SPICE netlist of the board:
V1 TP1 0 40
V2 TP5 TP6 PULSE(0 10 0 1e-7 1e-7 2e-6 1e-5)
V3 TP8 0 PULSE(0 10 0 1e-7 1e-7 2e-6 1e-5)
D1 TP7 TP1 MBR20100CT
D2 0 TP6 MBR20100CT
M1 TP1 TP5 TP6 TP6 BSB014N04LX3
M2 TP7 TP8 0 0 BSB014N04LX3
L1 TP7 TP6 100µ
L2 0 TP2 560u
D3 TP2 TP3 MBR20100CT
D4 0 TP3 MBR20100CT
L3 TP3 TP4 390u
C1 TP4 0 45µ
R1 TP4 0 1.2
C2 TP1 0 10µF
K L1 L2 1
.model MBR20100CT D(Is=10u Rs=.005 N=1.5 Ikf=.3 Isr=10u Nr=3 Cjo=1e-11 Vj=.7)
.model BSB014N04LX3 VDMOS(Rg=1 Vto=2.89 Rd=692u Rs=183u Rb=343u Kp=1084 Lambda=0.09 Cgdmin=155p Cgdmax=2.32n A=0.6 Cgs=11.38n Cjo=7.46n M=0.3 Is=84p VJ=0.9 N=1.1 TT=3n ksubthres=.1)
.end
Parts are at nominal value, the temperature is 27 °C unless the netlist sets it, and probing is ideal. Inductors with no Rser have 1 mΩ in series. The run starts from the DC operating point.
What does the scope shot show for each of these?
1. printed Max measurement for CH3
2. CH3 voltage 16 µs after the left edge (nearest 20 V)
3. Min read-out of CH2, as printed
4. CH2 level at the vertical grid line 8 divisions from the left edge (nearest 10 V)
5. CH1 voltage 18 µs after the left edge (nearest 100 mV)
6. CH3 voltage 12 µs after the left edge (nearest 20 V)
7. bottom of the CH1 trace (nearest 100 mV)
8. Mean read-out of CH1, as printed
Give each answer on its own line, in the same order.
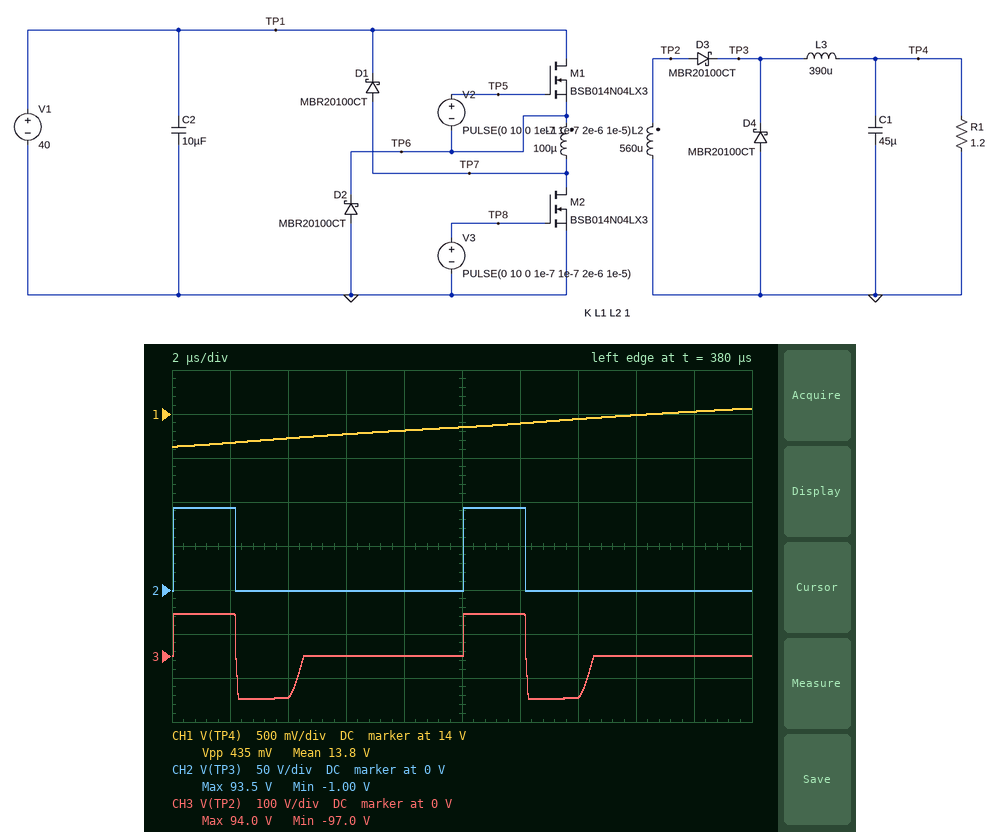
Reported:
94.0 V
0 V
-1.00 V
0 V
14.0 V
100 V
13.6 V
13.8 V
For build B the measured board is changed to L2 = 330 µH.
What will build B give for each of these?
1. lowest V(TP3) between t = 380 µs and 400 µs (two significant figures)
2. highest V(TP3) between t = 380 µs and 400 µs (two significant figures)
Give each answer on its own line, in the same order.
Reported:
-720 mV
72 V
